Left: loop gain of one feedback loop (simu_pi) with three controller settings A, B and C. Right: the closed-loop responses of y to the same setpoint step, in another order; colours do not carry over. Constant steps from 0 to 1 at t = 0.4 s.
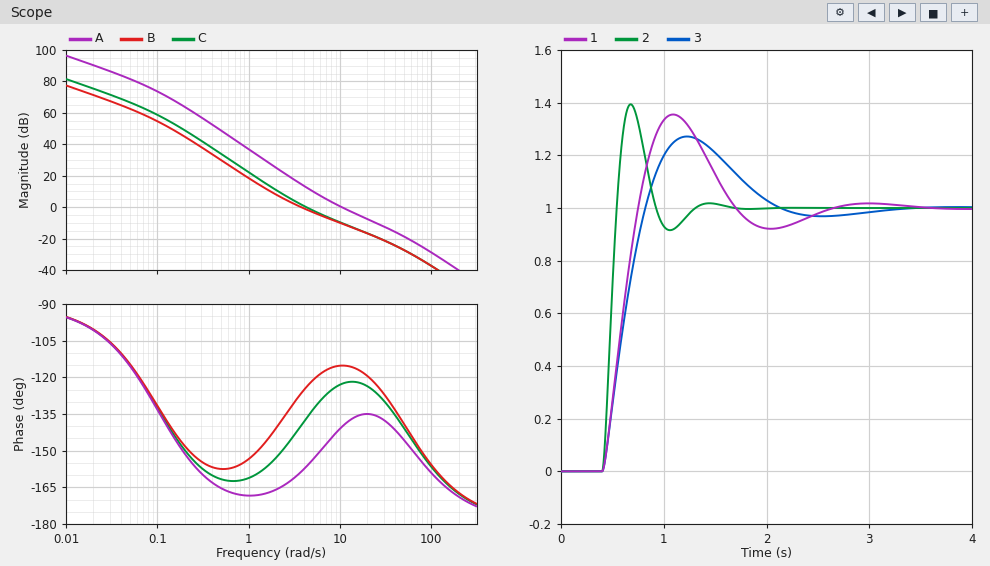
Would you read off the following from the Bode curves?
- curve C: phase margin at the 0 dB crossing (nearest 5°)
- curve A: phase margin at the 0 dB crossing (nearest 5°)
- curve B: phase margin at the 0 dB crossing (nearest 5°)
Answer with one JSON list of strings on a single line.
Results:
["45°", "40°", "55°"]
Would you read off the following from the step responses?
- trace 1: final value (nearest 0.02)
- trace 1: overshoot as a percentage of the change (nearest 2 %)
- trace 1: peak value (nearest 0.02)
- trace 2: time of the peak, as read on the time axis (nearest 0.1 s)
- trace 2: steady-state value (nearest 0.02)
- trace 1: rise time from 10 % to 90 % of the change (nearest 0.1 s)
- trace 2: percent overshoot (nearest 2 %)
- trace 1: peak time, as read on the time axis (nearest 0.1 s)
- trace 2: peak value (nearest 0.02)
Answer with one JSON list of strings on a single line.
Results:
["1.00", "36 %", "1.36", "0.7 s", "1.00", "0.3 s", "40 %", "1.1 s", "1.40"]
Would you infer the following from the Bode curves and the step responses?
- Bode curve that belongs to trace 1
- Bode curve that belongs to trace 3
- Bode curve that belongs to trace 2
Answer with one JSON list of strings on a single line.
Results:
["C", "B", "A"]
